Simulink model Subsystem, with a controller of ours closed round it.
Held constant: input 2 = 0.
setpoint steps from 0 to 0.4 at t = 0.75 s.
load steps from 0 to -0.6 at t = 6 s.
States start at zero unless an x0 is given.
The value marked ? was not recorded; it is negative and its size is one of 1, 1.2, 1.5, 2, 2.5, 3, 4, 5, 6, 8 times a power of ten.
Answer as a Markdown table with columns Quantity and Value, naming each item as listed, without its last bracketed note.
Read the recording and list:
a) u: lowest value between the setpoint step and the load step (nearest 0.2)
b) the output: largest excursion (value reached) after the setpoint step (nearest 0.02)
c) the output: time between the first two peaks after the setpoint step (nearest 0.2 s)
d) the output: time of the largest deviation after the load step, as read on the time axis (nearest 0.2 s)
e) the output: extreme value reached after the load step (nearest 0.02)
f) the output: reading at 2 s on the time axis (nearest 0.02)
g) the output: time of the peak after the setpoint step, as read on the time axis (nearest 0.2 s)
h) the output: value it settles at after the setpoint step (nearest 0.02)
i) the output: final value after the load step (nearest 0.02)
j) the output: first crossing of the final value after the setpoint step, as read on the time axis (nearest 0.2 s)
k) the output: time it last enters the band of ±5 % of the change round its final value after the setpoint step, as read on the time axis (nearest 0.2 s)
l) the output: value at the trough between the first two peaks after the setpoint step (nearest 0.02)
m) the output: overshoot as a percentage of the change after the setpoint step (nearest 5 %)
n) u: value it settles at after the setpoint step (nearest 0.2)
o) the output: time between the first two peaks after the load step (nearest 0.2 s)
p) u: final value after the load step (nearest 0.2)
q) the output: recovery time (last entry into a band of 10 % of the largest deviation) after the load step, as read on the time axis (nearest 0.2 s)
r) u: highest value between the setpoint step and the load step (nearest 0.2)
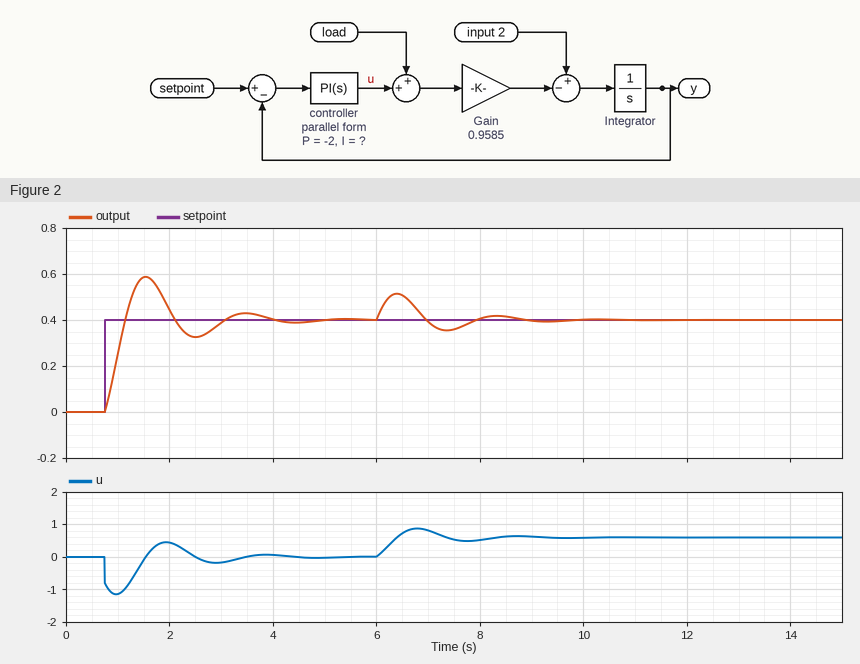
| Quantity | Value |
|---|---|
| u: lowest value between the setpoint step and the load step | -1.2 |
| the output: largest excursion (value reached) after the setpoint step | 0.58 |
| the output: time between the first two peaks after the setpoint step | 2.0 s |
| the output: time of the largest deviation after the load step, as read on the time axis | 6.4 s |
| the output: extreme value reached after the load step | 0.52 |
| the output: reading at 2 s on the time axis | 0.44 |
| the output: time of the peak after the setpoint step, as read on the time axis | 1.6 s |
| the output: value it settles at after the setpoint step | 0.40 |
| the output: final value after the load step | 0.40 |
| the output: first crossing of the final value after the setpoint step, as read on the time axis | 1.2 s |
| the output: time it last enters the band of ±5 % of the change round its final value after the setpoint step, as read on the time axis | 3.8 s |
| the output: value at the trough between the first two peaks after the setpoint step | 0.32 |
| the output: overshoot as a percentage of the change after the setpoint step | 45 % |
| u: value it settles at after the setpoint step | 0.0 |
| the output: time between the first two peaks after the load step | 2.0 s |
| u: final value after the load step | 0.6 |
| the output: recovery time (last entry into a band of 10 % of the largest deviation) after the load step, as read on the time axis | 8.6 s |
| u: highest value between the setpoint step and the load step | 0.4 |
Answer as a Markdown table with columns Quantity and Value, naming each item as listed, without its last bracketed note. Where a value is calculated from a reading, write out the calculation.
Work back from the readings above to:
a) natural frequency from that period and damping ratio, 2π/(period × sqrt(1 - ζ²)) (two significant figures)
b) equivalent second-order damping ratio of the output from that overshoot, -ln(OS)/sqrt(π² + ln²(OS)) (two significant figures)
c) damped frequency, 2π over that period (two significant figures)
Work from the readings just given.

| Quantity | Value |
|---|---|
| natural frequency from that period and damping ratio, 2π/(period × sqrt(1 - ζ²)) | 2π / (2 × sqrt(1 - 0.25²)) = 3.2 rad/s |
| equivalent second-order damping ratio of the output from that overshoot, -ln(OS)/sqrt(π² + ln²(OS)) | ln(0.45) = -0.799; 0.799 / sqrt(9.870 + 0.638) = 0.25 |
| damped frequency, 2π over that period | 2π / 2 = 3.1 rad/s |
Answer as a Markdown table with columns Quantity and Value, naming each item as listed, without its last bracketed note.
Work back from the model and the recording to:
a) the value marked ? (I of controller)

| Quantity | Value |
|---|---|
| the value marked ? | -12 |
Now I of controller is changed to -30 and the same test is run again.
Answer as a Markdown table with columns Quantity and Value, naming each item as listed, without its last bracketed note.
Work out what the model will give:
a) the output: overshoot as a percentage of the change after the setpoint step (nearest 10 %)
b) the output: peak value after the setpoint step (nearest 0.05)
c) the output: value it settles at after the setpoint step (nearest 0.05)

| Quantity | Value |
|---|---|
| the output: overshoot as a percentage of the change after the setpoint step | 60 % |
| the output: peak value after the setpoint step | 0.65 |
| the output: value it settles at after the setpoint step | 0.40 |
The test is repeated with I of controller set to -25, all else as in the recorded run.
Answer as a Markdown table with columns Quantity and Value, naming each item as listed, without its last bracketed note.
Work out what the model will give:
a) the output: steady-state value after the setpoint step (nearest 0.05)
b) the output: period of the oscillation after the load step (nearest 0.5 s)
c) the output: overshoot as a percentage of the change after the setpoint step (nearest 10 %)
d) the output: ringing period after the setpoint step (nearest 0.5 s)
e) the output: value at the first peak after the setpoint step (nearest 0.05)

| Quantity | Value |
|---|---|
| the output: steady-state value after the setpoint step | 0.40 |
| the output: period of the oscillation after the load step | 1.5 s |
| the output: overshoot as a percentage of the change after the setpoint step | 60 % |
| the output: ringing period after the setpoint step | 1.5 s |
| the output: value at the first peak after the setpoint step | 0.65 |
